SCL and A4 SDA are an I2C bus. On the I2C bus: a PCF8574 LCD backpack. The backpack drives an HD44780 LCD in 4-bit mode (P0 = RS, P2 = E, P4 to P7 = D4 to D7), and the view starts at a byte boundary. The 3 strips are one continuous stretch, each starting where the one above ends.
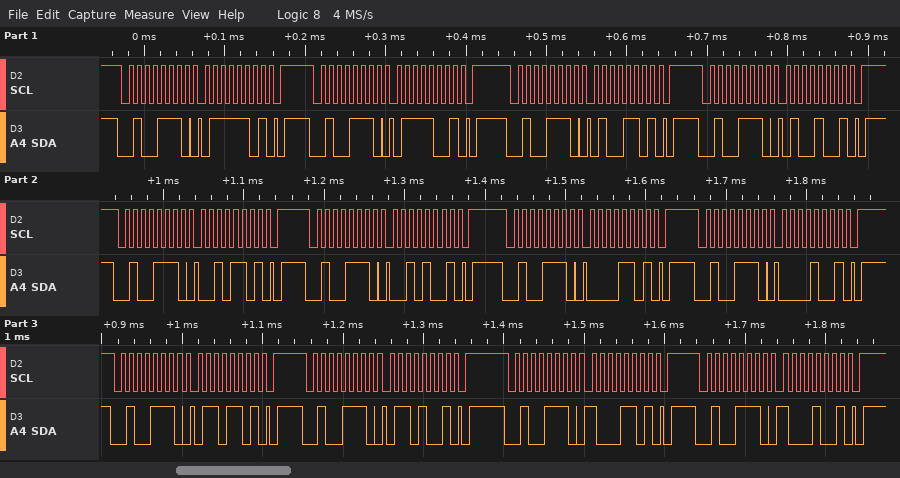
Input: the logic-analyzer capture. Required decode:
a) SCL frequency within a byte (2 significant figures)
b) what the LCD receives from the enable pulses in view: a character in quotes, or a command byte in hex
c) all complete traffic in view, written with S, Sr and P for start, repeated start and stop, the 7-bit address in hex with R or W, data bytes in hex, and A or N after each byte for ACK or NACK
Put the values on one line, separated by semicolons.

100 kHz; 't' ' ' 'h'; S 27W A 7D A P S 27W A 79 A P S 27W A 4D A P S 27W A 49 A P S 27W A 2D A P S 27W A 29 A P S 27W A 0D A P S 27W A 09 A P S 27W A 6D A P S 27W A 69 A P S 27W A 8D A P S 27W A 89 A P
